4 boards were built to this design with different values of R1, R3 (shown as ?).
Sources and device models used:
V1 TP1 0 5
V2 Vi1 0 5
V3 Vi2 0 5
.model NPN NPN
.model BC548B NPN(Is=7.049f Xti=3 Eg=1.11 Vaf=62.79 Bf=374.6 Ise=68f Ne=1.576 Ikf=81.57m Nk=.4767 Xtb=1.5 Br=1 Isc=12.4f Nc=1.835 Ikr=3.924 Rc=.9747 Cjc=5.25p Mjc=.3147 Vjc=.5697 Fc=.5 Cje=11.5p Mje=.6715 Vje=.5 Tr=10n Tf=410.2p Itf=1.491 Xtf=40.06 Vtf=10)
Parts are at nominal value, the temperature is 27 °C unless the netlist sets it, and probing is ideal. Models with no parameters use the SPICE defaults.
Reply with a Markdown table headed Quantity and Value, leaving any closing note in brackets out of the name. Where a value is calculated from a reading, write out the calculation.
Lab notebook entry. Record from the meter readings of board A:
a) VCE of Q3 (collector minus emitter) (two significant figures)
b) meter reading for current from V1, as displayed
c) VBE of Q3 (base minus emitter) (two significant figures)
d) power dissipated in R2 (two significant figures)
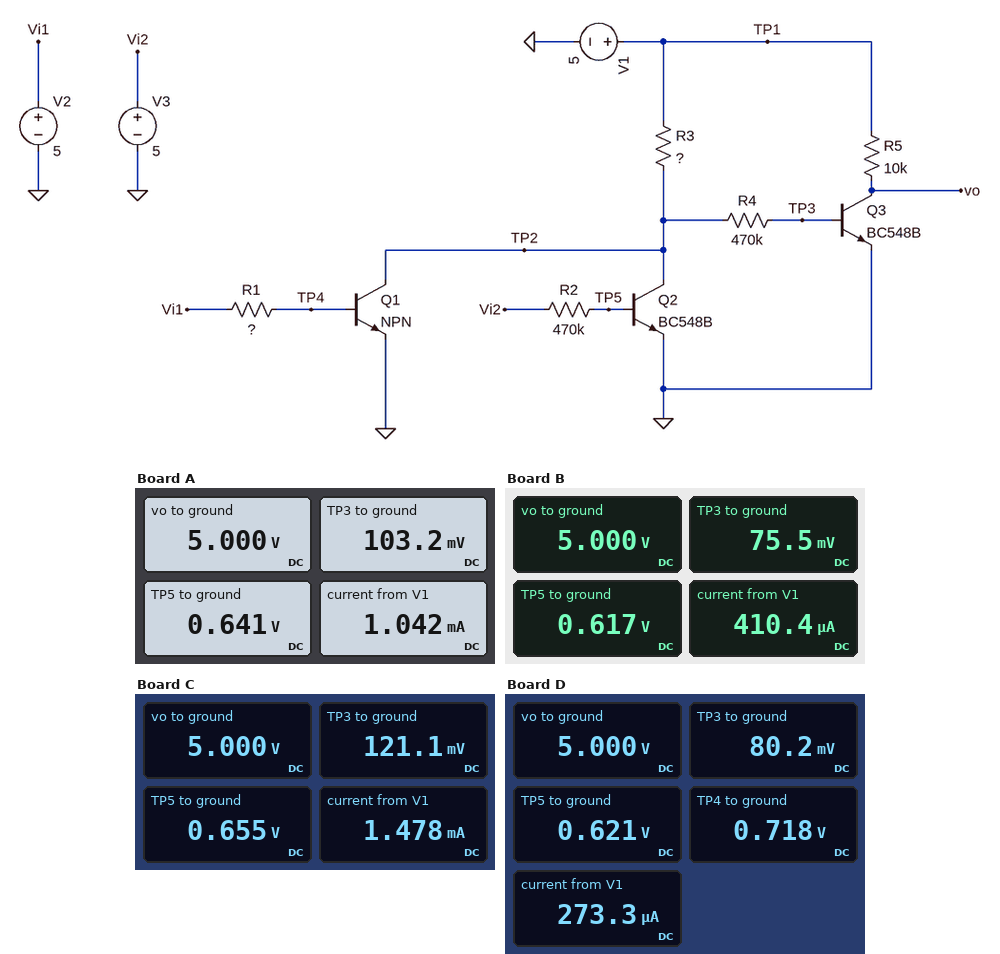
| Quantity | Value |
|---|---|
| VCE of Q3 (collector minus emitter) | 5 V = 5.0 V |
| meter reading for current from V1, as displayed | 1.042 mA |
| VBE of Q3 (base minus emitter) | 103.2 mV = 100 mV |
| power dissipated in R2 | (5 V - 641 mV)^2 / 470 kΩ = 40 µW |
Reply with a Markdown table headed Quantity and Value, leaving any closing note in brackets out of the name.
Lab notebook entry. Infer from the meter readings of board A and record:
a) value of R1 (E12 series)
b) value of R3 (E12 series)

| Quantity | Value |
|---|---|
| value of R1 | 220 kΩ |
| value of R3 | 4.7 kΩ |
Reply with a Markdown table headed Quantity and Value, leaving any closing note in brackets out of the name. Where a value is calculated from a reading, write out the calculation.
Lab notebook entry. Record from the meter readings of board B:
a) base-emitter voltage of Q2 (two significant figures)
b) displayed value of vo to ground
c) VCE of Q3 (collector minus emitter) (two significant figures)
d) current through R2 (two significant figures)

| Quantity | Value |
|---|---|
| base-emitter voltage of Q2 | 617 mV = 620 mV |
| displayed value of vo to ground | 5.000 V |
| VCE of Q3 (collector minus emitter) | 5 V = 5.0 V |
| current through R2 | (5 V - 617 mV) / 470 kΩ = 9.3 µA |
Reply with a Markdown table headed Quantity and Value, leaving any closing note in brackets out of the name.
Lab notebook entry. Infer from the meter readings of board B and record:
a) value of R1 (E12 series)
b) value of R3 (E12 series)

| Quantity | Value |
|---|---|
| value of R1 | 220 kΩ |
| value of R3 | 12 kΩ |
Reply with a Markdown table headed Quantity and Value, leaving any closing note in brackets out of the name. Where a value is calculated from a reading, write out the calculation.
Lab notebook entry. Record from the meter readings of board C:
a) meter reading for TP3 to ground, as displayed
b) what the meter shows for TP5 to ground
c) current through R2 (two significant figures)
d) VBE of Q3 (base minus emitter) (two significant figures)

| Quantity | Value |
|---|---|
| meter reading for TP3 to ground, as displayed | 121.1 mV |
| what the meter shows for TP5 to ground | 0.655 V |
| current through R2 | (5 V - 655 mV) / 470 kΩ = 9.2 µA |
| VBE of Q3 (base minus emitter) | 121.1 mV = 120 mV |
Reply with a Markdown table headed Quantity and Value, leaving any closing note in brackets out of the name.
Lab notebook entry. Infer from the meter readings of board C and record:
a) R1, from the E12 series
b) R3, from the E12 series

| Quantity | Value |
|---|---|
| R1, from the E12 series | 270 kΩ |
| R3, from the E12 series | 3.3 kΩ |
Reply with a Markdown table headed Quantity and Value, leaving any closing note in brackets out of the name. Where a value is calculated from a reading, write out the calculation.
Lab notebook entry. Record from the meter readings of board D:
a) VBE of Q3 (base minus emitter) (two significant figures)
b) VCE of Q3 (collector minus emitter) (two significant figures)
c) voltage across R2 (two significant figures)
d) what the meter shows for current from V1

| Quantity | Value |
|---|---|
| VBE of Q3 (base minus emitter) | 80.2 mV = 80 mV |
| VCE of Q3 (collector minus emitter) | 5 V = 5.0 V |
| voltage across R2 | 5 V - 621 mV = 4.4 V |
| what the meter shows for current from V1 | 273.3 µA |
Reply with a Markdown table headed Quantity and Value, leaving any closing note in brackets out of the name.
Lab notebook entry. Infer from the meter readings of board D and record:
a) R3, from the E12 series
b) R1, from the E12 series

| Quantity | Value |
|---|---|
| R3, from the E12 series | 18 kΩ |
| R1, from the E12 series | 680 kΩ |
